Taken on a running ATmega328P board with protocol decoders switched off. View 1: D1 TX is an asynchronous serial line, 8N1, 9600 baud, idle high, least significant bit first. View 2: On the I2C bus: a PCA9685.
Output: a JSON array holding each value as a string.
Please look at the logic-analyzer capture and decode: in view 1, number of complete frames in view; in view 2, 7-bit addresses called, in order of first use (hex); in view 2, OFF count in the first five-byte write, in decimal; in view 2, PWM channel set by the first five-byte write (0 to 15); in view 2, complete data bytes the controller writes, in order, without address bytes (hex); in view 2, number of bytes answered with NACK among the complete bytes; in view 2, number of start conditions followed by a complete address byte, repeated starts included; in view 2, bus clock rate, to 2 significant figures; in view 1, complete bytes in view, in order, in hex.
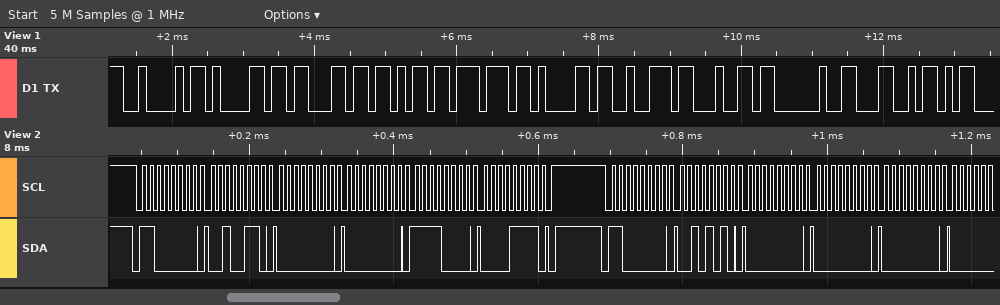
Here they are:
["10", "0x60", "4080", "8", "26 00 00 F0 0F 2A 00 00 00", "0", "2", "100 kHz", "42 61 63 6B 77 61 72 64 20 4C"]
